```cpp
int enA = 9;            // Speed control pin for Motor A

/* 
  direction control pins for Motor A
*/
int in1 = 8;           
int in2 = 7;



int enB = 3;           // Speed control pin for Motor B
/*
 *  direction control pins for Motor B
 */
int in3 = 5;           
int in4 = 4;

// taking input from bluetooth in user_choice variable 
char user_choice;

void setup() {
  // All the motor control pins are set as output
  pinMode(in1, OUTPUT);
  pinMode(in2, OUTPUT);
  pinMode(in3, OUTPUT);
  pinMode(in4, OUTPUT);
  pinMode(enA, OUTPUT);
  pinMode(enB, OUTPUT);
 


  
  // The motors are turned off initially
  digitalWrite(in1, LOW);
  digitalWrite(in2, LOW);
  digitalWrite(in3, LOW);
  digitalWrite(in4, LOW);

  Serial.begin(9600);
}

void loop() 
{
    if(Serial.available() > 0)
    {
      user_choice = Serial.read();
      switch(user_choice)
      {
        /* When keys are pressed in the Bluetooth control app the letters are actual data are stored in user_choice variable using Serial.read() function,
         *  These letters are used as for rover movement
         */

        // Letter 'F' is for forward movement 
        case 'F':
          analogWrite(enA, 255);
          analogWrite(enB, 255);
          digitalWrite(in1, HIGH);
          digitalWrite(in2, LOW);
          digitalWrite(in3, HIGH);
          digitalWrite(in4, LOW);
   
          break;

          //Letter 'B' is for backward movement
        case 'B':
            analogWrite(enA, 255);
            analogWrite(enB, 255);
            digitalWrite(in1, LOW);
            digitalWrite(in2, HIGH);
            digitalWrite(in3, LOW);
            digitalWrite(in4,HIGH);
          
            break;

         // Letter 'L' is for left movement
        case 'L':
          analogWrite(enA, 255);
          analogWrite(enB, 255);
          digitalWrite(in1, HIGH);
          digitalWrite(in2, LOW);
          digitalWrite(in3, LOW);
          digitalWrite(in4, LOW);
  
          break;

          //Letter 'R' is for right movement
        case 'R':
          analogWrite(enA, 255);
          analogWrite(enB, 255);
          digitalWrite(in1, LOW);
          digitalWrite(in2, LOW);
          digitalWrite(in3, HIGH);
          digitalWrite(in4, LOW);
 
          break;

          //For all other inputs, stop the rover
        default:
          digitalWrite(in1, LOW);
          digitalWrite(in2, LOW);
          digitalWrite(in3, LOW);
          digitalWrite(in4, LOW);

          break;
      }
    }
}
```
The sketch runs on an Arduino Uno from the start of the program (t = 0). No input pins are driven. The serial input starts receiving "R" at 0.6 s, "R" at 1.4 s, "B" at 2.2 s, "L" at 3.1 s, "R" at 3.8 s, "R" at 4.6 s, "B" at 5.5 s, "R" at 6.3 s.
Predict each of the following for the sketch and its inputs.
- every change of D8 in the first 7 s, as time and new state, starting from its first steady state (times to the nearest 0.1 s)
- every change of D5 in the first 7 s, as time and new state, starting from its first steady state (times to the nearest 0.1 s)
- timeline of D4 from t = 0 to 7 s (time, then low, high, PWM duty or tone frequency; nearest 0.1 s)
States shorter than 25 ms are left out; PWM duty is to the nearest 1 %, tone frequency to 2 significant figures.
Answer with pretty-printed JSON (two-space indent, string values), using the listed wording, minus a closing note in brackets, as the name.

{
  "every change of D8 in the first 7 s, as time and new state, starting from its first steady state": "0 s low; 3.1 s high; 3.8 s low",
  "every change of D5 in the first 7 s, as time and new state, starting from its first steady state": "0 s low; 0.6 s high; 2.2 s low; 3.8 s high; 5.5 s low; 6.3 s high",
  "timeline of D4 from t = 0 to 7 s": "0 s low; 2.2 s high; 3.1 s low; 5.5 s high; 6.3 s low"
}
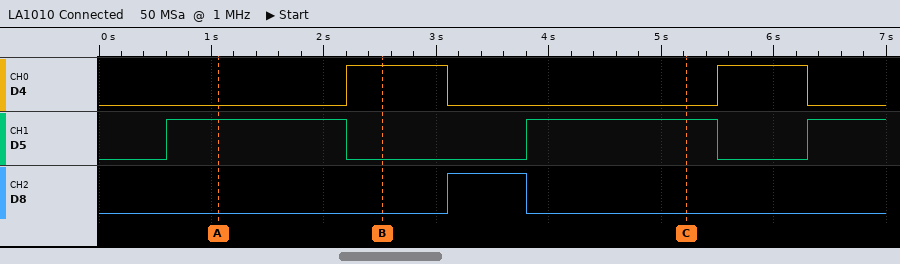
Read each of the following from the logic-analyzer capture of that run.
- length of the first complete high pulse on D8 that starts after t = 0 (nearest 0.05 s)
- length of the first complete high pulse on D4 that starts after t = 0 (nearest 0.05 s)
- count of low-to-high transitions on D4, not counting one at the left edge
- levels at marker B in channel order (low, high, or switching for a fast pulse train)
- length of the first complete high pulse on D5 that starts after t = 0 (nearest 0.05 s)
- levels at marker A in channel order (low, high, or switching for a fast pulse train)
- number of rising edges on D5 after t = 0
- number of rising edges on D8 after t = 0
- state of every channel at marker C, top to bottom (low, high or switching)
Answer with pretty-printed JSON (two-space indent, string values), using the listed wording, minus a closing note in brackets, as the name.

{
  "length of the first complete high pulse on D8 that starts after t = 0": "0.70 s",
  "length of the first complete high pulse on D4 that starts after t = 0": "0.90 s",
  "count of low-to-high transitions on D4, not counting one at the left edge": "2",
  "levels at marker B in channel order": "D4 high, D5 low, D8 low",
  "length of the first complete high pulse on D5 that starts after t = 0": "1.60 s",
  "levels at marker A in channel order": "D4 low, D5 high, D8 low",
  "number of rising edges on D5 after t = 0": "3",
  "number of rising edges on D8 after t = 0": "1",
  "state of every channel at marker C, top to bottom": "D4 low, D5 high, D8 low"
}
